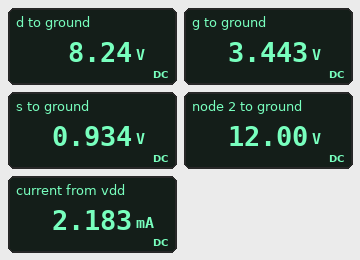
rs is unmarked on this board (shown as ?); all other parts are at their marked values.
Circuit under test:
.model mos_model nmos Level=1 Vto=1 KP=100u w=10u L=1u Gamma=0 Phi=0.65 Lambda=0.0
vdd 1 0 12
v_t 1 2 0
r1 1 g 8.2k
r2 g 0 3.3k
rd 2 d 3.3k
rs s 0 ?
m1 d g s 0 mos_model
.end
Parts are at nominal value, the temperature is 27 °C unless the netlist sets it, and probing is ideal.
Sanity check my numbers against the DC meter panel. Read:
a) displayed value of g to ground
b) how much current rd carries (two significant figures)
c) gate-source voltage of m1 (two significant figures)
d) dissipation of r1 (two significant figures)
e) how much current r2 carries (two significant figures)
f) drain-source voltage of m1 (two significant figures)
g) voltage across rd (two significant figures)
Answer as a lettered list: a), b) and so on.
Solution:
a) 3.443 V
b) 1.1 mA
c) 2.5 V
d) 8.9 mW
e) 1.0 mA
f) 7.3 V
g) 3.8 V
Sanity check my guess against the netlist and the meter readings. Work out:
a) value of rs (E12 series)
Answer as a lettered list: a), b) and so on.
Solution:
a) 820 Ω
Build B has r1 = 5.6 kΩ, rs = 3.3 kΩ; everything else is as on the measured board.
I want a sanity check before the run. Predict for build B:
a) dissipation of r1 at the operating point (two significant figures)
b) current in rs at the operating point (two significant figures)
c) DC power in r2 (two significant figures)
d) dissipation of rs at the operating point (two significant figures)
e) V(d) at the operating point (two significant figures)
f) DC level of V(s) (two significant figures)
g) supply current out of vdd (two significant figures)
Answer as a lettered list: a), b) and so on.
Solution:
a) 10 mW
b) 690 µA
c) 6.0 mW
d) 1.6 mW
e) 9.7 V
f) 2.3 V
g) 2.0 mA
